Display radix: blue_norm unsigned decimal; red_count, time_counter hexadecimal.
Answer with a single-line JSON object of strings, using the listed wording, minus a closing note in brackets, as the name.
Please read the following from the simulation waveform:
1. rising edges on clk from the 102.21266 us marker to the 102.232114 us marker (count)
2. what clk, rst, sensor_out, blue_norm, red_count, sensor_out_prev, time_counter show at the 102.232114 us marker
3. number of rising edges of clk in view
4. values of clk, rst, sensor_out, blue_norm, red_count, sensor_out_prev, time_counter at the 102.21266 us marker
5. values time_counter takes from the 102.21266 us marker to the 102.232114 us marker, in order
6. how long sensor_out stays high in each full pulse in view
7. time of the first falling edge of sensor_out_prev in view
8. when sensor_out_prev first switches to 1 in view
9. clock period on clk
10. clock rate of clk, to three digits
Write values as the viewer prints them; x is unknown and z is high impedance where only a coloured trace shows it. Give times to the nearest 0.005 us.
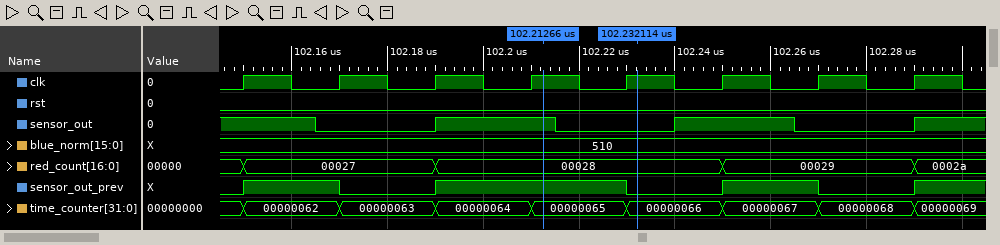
{"rising edges on clk from the 102.21266 us marker to the 102.232114 us marker": "1", "what clk, rst, sensor_out, blue_norm, red_count, sensor_out_prev, time_counter show at the 102.232114 us marker": "clk=1, rst=0, sensor_out=0, blue_norm=510, red_count=00028, sensor_out_prev=0, time_counter=00000066", "number of rising edges of clk in view": "8", "values of clk, rst, sensor_out, blue_norm, red_count, sensor_out_prev, time_counter at the 102.21266 us marker": "clk=1, rst=0, sensor_out=1, blue_norm=510, red_count=00028, sensor_out_prev=1, time_counter=00000065", "values time_counter takes from the 102.21266 us marker to the 102.232114 us marker, in order": "00000065, 00000066", "how long sensor_out stays high in each full pulse in view": "0.025 us, 0.025 us", "time of the first falling edge of sensor_out_prev in view": "102.17 us", "when sensor_out_prev first switches to 1 in view": "102.15 us", "clock period on clk": "0.02 us", "clock rate of clk, to three digits": "50.0 MHz"}
